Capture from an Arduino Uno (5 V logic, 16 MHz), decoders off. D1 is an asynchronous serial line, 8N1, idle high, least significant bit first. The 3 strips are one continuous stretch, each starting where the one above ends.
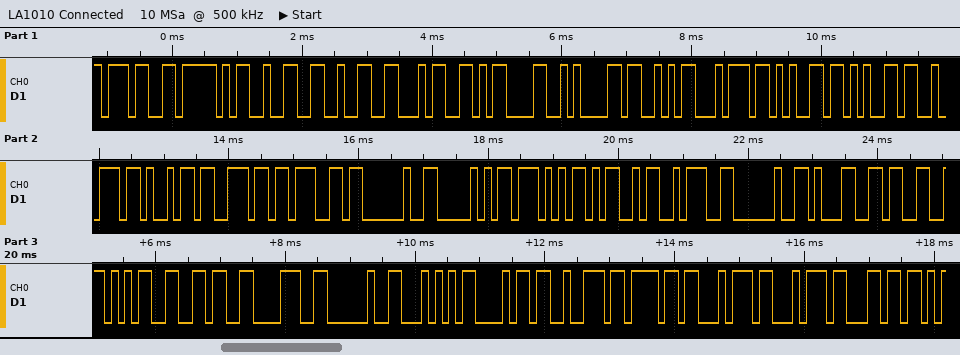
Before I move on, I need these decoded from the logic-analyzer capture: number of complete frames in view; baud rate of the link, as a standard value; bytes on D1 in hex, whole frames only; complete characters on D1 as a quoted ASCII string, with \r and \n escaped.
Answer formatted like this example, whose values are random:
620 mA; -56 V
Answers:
34; 9600 baud; 37 5F 32 32 34 0D 0A 53 74 65 65 72 69 6E 67 20 50 57 4D 3A 20 31 33 35 36 38 20 54 68 72 6F 74 74 6C; "7_224\r\nSteering PWM: 13568 Throttl"
